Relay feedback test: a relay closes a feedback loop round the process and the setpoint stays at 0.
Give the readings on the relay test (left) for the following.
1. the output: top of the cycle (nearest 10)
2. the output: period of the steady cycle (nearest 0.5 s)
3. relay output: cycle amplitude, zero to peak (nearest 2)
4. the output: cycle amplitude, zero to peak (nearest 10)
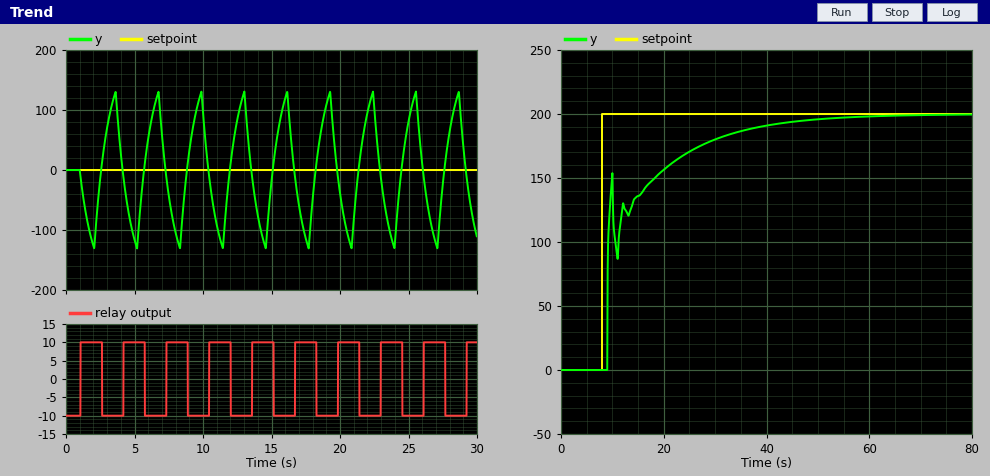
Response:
130
3.0 s
10
130
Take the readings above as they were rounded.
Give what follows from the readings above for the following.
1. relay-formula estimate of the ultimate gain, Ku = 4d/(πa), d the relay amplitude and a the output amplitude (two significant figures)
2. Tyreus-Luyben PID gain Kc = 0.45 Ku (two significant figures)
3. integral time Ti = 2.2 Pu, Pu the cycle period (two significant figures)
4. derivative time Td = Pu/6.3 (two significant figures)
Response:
0.098
0.044
6.6 s
0.48 s
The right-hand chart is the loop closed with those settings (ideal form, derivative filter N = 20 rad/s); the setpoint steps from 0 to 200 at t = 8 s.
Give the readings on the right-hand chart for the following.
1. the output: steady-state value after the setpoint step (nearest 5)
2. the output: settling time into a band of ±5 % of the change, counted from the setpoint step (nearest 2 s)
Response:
200
30 s
